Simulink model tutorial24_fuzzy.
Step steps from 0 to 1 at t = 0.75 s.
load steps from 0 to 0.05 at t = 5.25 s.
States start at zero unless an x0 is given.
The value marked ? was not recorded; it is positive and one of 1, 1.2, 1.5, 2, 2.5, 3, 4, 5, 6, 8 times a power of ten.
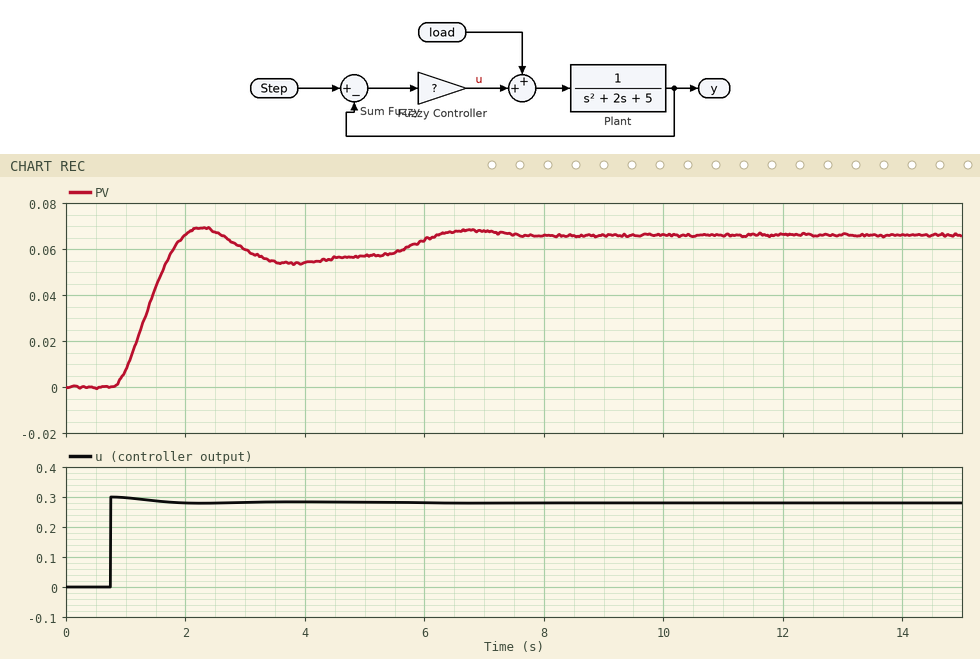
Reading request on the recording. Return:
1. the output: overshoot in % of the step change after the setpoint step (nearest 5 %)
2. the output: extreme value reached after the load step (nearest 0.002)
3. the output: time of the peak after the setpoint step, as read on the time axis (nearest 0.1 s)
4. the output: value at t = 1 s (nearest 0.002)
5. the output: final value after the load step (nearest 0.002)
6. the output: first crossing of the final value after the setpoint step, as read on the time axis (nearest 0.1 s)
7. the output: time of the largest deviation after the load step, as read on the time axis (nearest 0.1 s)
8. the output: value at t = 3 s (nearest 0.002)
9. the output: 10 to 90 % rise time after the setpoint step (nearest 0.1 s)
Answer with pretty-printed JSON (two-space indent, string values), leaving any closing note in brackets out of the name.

{
  "the output: overshoot in % of the step change after the setpoint step": "20 %",
  "the output: extreme value reached after the load step": "0.068",
  "the output: time of the peak after the setpoint step, as read on the time axis": "2.3 s",
  "the output: value at t = 1 s": "0.008",
  "the output: final value after the load step": "0.066",
  "the output: first crossing of the final value after the setpoint step, as read on the time axis": "1.7 s",
  "the output: time of the largest deviation after the load step, as read on the time axis": "6.8 s",
  "the output: value at t = 3 s": "0.060",
  "the output: 10 to 90 % rise time after the setpoint step": "0.7 s"
}
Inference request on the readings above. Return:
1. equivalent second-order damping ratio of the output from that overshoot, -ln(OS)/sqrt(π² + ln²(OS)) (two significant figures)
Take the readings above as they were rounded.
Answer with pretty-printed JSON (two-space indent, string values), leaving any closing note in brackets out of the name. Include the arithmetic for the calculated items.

{
  "equivalent second-order damping ratio of the output from that overshoot, -ln(OS)/sqrt(π² + ln²(OS))": "ln(0.2) = -1.609; 1.609 / sqrt(9.870 + 2.590) = 0.46"
}
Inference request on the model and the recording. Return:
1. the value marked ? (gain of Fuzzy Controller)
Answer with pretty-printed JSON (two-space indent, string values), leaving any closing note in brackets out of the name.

{
  "the value marked ?": "0.3"
}
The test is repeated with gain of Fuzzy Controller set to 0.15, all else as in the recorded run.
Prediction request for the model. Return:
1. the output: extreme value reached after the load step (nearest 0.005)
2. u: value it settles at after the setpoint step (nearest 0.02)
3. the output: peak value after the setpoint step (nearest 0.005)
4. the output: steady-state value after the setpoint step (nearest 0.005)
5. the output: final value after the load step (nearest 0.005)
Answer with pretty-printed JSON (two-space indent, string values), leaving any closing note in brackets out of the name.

{
  "the output: extreme value reached after the load step": "0.040",
  "u: value it settles at after the setpoint step": "0.14",
  "the output: peak value after the setpoint step": "0.035",
  "the output: steady-state value after the setpoint step": "0.030",
  "the output: final value after the load step": "0.040"
}
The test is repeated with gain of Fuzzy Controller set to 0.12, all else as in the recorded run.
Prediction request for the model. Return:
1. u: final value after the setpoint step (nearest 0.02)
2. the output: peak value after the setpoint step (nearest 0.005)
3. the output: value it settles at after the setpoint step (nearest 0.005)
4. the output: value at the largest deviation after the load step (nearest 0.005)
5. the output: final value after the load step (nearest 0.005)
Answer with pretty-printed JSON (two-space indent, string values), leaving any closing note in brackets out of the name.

{
  "u: final value after the setpoint step": "0.12",
  "the output: peak value after the setpoint step": "0.030",
  "the output: value it settles at after the setpoint step": "0.025",
  "the output: value at the largest deviation after the load step": "0.035",
  "the output: final value after the load step": "0.035"
}
